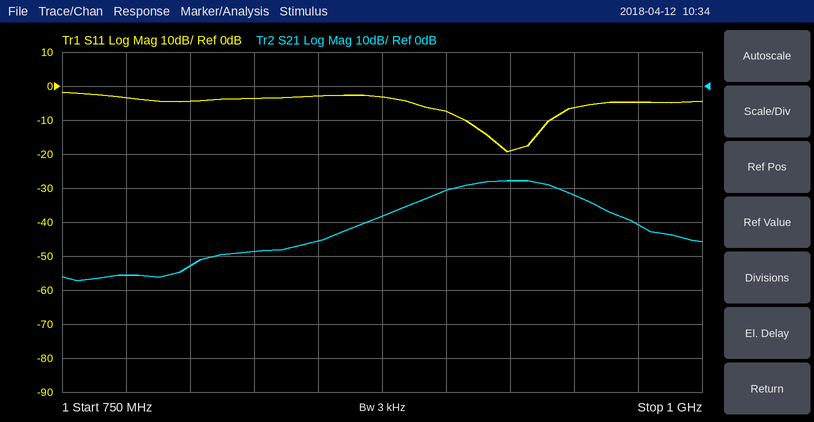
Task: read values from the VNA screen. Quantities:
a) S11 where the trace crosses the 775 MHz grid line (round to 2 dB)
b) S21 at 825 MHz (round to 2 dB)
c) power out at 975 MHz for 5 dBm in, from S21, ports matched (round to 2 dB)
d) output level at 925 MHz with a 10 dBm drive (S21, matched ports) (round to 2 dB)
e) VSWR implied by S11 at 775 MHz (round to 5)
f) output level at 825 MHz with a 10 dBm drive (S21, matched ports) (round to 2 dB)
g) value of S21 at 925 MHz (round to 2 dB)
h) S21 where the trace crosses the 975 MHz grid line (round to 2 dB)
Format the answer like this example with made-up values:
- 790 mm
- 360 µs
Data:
- -4 dB
- -48 dB
- -36 dBm
- -18 dBm
- 5
- -38 dBm
- -28 dB
- -40 dB
